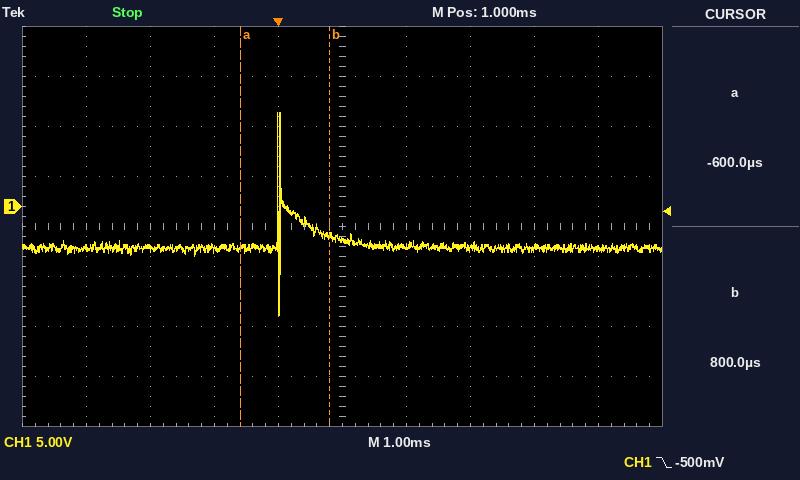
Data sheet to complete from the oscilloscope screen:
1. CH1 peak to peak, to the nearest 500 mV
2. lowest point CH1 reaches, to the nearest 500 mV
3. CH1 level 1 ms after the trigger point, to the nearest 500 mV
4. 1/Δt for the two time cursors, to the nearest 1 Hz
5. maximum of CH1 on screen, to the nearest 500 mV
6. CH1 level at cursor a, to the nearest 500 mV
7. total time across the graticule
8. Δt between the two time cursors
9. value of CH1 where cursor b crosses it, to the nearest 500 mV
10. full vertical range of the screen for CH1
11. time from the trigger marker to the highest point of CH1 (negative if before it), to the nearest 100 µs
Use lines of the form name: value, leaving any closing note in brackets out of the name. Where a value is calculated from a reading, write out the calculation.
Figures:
CH1 peak to peak, to the nearest 500 mV: 9.5 V − (-11.0 V) = 20.5 V
lowest point CH1 reaches, to the nearest 500 mV: -11.0 V
CH1 level 1 ms after the trigger point, to the nearest 500 mV: -3.5 V
1/Δt for the two time cursors, to the nearest 1 Hz: 1 / 1.4 ms ≈ 714 Hz
maximum of CH1 on screen, to the nearest 500 mV: 9.5 V
CH1 level at cursor a, to the nearest 500 mV: -4.0 V
total time across the graticule: 10 ms
Δt between the two time cursors: 800 µs − (-600 µs) = 1.4 ms
value of CH1 where cursor b crosses it, to the nearest 500 mV: -3.0 V
full vertical range of the screen for CH1: 40 V
time from the trigger marker to the highest point of CH1 (negative if before it), to the nearest 100 µs: 0.0 ms
